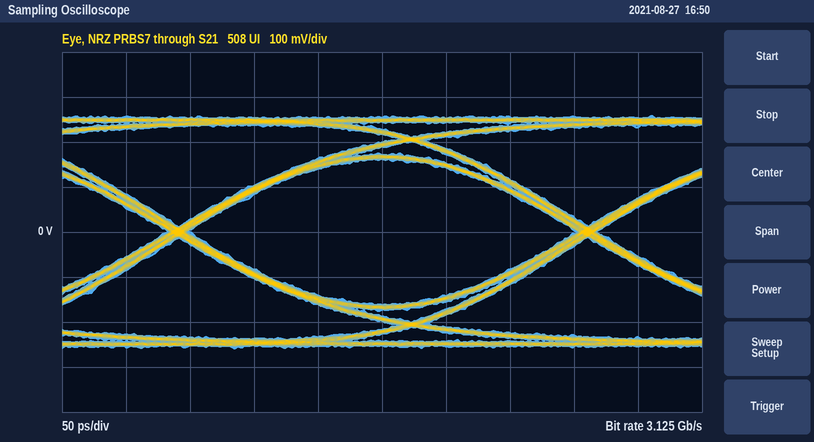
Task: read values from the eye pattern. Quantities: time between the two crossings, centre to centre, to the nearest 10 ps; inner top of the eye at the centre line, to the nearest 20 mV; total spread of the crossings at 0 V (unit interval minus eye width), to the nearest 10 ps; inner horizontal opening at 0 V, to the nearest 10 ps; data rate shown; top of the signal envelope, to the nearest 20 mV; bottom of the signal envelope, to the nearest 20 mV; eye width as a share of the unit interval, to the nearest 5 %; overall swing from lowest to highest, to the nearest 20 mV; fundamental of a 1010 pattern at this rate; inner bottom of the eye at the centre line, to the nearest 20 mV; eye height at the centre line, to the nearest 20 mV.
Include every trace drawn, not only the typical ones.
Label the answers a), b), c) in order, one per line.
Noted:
a) 320 ps
b) 160 mV
c) 20 ps
d) 300 ps
e) 3.125 Gb/s
f) 260 mV
g) -260 mV
h) 95 %
i) 520 mV
j) 1.5625 GHz
k) -160 mV
l) 320 mV
